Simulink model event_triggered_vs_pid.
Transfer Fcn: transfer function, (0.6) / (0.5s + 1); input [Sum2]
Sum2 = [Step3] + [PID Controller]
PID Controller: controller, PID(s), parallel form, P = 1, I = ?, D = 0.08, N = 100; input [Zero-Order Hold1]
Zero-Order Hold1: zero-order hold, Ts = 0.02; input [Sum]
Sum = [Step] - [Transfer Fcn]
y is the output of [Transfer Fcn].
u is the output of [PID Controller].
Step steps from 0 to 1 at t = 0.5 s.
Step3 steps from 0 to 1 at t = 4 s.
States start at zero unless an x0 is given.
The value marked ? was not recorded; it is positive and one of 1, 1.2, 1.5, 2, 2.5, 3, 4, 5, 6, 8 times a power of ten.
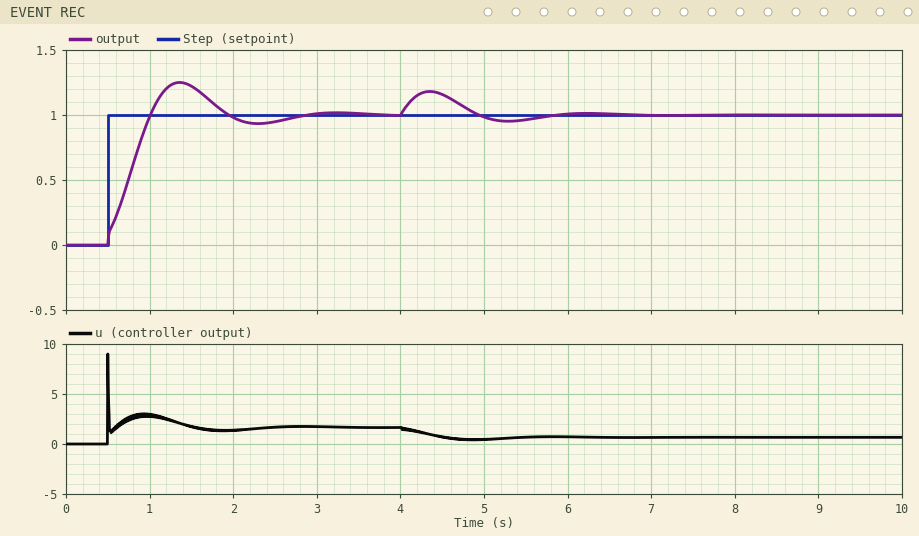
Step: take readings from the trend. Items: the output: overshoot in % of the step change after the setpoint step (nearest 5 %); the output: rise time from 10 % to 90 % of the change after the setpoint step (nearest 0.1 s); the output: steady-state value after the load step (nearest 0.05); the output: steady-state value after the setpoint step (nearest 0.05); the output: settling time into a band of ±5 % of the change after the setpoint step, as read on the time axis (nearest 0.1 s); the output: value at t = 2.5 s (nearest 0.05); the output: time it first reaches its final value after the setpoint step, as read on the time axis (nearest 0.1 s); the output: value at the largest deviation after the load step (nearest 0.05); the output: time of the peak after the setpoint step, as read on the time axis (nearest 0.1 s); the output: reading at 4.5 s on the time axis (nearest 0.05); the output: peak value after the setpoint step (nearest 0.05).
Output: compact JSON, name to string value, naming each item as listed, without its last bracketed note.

{"the output: overshoot in % of the step change after the setpoint step": "25 %", "the output: rise time from 10 % to 90 % of the change after the setpoint step": "0.4 s", "the output: steady-state value after the load step": "1.00", "the output: steady-state value after the setpoint step": "1.00", "the output: settling time into a band of ±5 % of the change after the setpoint step, as read on the time axis": "2.5 s", "the output: value at t = 2.5 s": "0.95", "the output: time it first reaches its final value after the setpoint step, as read on the time axis": "1.0 s", "the output: value at the largest deviation after the load step": "1.20", "the output: time of the peak after the setpoint step, as read on the time axis": "1.4 s", "the output: reading at 4.5 s on the time axis": "1.15", "the output: peak value after the setpoint step": "1.25"}
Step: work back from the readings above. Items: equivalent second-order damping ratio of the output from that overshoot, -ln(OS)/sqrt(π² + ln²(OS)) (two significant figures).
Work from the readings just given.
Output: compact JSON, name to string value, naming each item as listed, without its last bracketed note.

{"equivalent second-order damping ratio of the output from that overshoot, -ln(OS)/sqrt(π² + ln²(OS))": "0.40"}
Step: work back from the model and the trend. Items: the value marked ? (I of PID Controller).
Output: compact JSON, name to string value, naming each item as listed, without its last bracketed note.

{"the value marked ?": "12"}
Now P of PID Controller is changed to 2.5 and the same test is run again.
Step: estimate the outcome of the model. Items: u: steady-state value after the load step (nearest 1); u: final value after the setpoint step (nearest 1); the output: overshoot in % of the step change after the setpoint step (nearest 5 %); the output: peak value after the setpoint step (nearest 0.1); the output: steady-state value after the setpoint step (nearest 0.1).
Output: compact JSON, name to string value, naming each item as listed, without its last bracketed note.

{"u: steady-state value after the load step": "1", "u: final value after the setpoint step": "2", "the output: overshoot in % of the step change after the setpoint step": "10 %", "the output: peak value after the setpoint step": "1.1", "the output: steady-state value after the setpoint step": "1.0"}
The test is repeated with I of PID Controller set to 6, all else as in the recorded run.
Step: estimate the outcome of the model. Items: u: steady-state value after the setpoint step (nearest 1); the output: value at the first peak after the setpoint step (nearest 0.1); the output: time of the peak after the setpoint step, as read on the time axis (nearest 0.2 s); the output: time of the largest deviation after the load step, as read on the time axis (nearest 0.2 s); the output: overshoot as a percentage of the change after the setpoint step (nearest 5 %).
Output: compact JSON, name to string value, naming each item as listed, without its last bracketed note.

{"u: steady-state value after the setpoint step": "2", "the output: value at the first peak after the setpoint step": "1.1", "the output: time of the peak after the setpoint step, as read on the time axis": "1.8 s", "the output: time of the largest deviation after the load step, as read on the time axis": "4.4 s", "the output: overshoot as a percentage of the change after the setpoint step": "10 %"}
